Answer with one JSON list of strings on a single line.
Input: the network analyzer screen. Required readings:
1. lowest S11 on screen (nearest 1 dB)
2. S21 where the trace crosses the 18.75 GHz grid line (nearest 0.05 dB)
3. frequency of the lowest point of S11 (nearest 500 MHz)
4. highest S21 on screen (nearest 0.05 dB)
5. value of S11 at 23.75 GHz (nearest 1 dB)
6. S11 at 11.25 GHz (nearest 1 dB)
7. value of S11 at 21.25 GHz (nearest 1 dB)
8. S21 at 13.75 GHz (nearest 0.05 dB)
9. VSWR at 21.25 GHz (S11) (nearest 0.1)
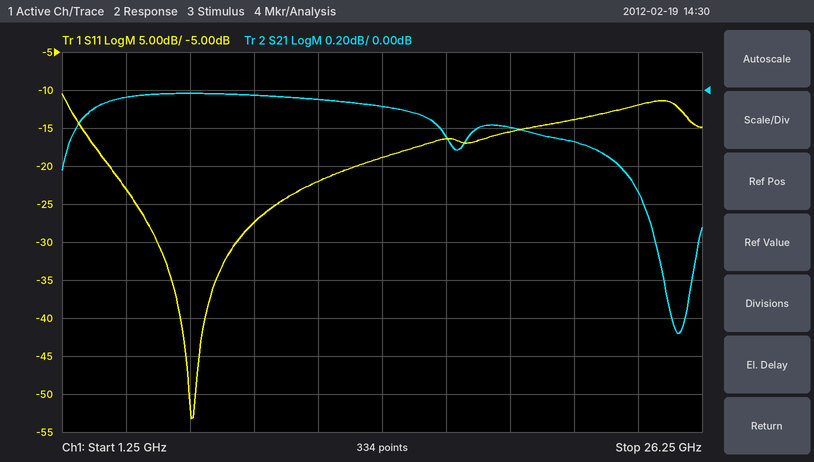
["-53 dB", "-0.20 dB", "6.5 GHz", "0.00 dB", "-12 dB", "-22 dB", "-14 dB", "-0.10 dB", "1.5"]
